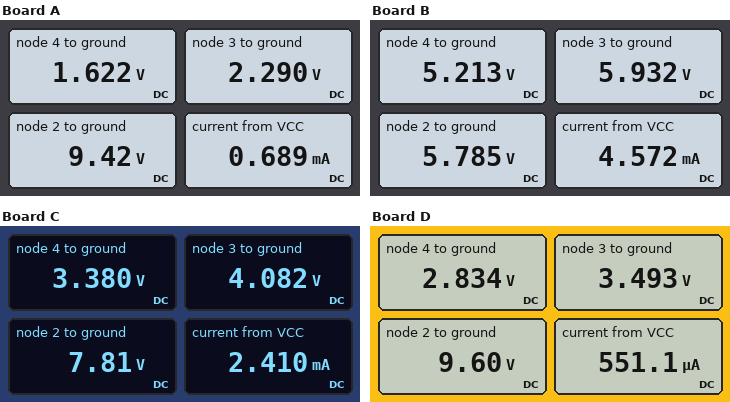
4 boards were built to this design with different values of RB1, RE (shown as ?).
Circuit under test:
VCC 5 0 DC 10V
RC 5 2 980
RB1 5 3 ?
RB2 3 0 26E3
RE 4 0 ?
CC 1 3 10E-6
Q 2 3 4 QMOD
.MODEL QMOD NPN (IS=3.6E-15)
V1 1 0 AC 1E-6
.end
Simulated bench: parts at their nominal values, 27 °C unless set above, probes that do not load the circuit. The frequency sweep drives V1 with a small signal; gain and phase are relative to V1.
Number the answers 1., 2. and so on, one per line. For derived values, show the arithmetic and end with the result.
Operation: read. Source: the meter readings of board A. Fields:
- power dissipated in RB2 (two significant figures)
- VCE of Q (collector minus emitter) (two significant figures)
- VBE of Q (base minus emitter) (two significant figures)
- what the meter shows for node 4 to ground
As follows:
1. (2.29 V)^2 / 26 kΩ = 200 µW
2. 9.42 V - 1.622 V = 7.8 V
3. 2.29 V - 1.622 V = 670 mV
4. 1.622 V
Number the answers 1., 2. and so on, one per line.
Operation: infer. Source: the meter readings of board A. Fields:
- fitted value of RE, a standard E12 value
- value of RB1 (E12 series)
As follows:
1. 2.7 kΩ
2. 82 kΩ
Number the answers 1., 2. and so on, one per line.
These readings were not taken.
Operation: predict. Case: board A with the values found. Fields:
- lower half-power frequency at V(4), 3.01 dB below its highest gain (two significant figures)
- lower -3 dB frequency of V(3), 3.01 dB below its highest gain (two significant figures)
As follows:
1. 860 mHz
2. 860 mHz
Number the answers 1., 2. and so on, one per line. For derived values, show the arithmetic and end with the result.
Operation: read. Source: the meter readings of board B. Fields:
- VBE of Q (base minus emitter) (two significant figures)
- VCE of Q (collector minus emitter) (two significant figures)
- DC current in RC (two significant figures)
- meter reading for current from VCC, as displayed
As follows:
1. 5.932 V - 5.213 V = 720 mV
2. 5.785 V - 5.213 V = 570 mV
3. (10 V - 5.785 V) / 980 Ω = 4.3 mA
4. 4.572 mA
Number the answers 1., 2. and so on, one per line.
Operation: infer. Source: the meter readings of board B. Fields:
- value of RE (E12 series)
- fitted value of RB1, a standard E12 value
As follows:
1. 1.2 kΩ
2. 15 kΩ
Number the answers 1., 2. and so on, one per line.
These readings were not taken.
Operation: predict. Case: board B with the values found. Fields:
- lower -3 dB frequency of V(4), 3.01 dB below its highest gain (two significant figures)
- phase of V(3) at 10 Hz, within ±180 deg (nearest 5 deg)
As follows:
1. 1.8 Hz
2. 10 deg
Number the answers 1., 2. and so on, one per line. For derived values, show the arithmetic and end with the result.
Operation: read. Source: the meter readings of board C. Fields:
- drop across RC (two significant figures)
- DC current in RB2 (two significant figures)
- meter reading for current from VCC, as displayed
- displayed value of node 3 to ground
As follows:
1. 10 V - 7.81 V = 2.2 V
2. (4.082 V) / 26 kΩ = 160 µA
3. 2.410 mA
4. 4.082 V
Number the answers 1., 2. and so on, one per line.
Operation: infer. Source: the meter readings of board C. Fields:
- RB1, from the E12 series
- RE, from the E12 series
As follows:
1. 33 kΩ
2. 1.5 kΩ
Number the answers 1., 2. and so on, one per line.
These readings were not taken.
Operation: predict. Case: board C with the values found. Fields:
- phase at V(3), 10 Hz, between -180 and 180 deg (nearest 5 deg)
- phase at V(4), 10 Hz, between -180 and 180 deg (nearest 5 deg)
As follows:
1. 5 deg
2. 5 deg
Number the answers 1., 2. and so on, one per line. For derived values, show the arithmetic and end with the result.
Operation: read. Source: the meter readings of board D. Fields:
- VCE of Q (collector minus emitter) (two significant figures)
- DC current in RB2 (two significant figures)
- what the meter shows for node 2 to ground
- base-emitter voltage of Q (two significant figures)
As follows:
1. 9.6 V - 2.834 V = 6.8 V
2. (3.493 V) / 26 kΩ = 130 µA
3. 9.60 V
4. 3.493 V - 2.834 V = 660 mV
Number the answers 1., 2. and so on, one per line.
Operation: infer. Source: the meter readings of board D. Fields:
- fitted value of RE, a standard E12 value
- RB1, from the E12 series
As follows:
1. 6.8 kΩ
2. 47 kΩ
